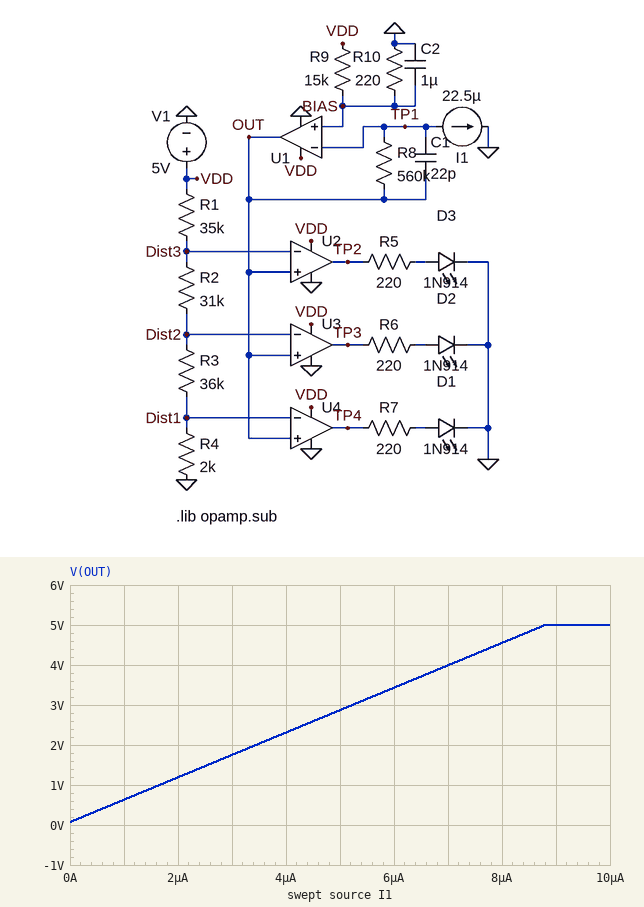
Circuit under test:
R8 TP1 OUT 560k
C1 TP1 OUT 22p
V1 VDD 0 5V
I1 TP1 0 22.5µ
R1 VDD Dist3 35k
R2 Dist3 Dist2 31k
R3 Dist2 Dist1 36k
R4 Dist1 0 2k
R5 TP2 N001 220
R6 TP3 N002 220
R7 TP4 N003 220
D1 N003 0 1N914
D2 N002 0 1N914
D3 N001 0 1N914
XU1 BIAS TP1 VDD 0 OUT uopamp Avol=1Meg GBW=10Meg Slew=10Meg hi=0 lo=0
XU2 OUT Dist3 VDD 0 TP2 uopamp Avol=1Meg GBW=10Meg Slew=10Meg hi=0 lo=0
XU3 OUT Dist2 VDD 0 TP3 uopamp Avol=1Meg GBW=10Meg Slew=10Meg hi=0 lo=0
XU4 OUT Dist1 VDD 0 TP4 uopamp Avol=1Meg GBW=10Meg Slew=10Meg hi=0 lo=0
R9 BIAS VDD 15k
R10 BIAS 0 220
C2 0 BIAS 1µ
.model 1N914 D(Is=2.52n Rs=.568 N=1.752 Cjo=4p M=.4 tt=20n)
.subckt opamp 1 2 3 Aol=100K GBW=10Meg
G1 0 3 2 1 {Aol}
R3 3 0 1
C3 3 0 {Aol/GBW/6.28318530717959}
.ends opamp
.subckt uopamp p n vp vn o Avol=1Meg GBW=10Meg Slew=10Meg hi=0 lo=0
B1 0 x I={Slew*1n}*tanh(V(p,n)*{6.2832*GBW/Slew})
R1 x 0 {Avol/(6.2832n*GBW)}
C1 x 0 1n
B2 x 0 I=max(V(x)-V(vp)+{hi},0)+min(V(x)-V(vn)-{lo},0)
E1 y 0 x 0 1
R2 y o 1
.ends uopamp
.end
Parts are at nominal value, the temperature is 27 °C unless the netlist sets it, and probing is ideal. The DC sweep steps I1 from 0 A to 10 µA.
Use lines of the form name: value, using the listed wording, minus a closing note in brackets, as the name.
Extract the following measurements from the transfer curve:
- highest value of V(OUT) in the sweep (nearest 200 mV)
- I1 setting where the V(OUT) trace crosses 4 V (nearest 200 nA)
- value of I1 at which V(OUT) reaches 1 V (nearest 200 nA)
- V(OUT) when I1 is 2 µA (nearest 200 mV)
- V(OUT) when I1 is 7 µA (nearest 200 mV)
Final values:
highest value of V(OUT) in the sweep: 5.0 V
I1 setting where the V(OUT) trace crosses 4 V: 7.0 µA
value of I1 at which V(OUT) reaches 1 V: 1.6 µA
V(OUT) when I1 is 2 µA: 1.2 V
V(OUT) when I1 is 7 µA: 4.0 V
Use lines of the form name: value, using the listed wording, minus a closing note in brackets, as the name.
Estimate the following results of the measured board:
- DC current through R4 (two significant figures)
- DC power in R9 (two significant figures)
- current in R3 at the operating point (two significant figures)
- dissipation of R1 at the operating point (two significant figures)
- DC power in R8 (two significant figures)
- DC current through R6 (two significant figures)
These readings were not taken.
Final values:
DC current through R4: 48 µA
DC power in R9: 1.6 mW
current in R3 at the operating point: 48 µA
dissipation of R1 at the operating point: 81 µW
DC power in R8: 280 µW
DC current through R6: 19 mA
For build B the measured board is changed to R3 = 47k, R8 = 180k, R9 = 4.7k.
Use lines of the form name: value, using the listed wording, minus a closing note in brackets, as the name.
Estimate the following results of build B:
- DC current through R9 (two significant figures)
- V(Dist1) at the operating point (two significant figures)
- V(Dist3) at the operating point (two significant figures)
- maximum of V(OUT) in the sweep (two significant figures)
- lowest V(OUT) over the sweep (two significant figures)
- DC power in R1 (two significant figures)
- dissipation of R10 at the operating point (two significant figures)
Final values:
DC current through R9: 1.0 mA
V(Dist1) at the operating point: 87 mV
V(Dist3) at the operating point: 3.5 V
maximum of V(OUT) in the sweep: 2.0 V
lowest V(OUT) over the sweep: 220 mV
DC power in R1: 66 µW
dissipation of R10 at the operating point: 230 µW
